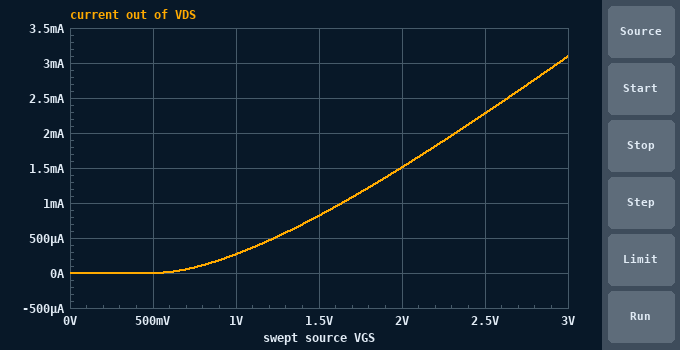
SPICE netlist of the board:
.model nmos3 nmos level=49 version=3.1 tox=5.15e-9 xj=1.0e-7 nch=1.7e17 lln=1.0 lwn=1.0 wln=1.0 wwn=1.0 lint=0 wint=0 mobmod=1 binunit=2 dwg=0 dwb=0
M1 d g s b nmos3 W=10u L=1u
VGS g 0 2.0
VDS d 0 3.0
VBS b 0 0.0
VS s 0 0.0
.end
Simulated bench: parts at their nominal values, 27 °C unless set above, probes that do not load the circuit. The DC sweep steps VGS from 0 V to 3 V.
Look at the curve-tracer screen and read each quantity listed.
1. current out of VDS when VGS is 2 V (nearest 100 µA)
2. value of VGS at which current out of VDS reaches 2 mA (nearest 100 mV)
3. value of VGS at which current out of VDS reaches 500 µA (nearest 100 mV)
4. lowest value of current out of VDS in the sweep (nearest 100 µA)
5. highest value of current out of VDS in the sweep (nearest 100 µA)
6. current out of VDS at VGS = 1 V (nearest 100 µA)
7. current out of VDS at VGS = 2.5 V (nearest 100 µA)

1.5 mA
2.3 V
1.2 V
0 A
3.1 mA
300 µA
2.3 mA
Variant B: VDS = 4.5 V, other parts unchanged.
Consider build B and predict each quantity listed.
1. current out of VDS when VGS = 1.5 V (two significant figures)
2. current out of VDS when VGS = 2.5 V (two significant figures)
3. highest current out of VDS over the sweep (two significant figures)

1.2 mA
2.8 mA
3.5 mA
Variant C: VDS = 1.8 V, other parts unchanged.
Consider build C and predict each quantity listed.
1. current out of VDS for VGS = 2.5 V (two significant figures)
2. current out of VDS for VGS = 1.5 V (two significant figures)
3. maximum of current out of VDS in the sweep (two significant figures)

2.2 mA
790 µA
3.0 mA
